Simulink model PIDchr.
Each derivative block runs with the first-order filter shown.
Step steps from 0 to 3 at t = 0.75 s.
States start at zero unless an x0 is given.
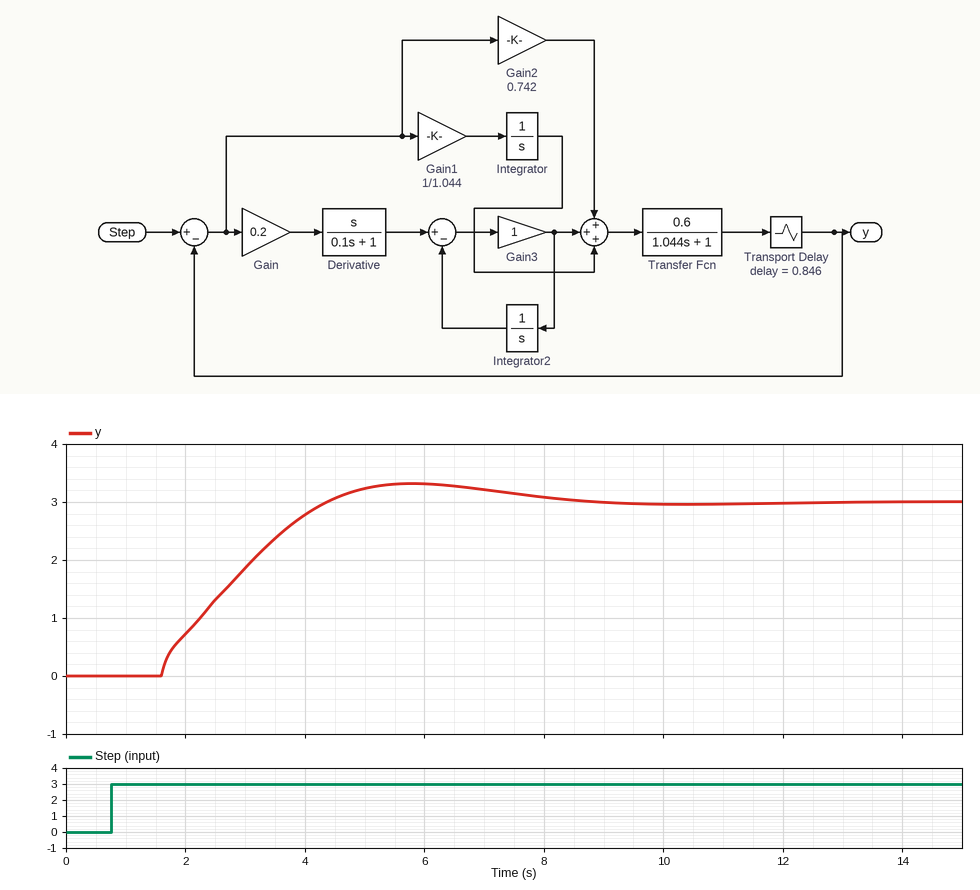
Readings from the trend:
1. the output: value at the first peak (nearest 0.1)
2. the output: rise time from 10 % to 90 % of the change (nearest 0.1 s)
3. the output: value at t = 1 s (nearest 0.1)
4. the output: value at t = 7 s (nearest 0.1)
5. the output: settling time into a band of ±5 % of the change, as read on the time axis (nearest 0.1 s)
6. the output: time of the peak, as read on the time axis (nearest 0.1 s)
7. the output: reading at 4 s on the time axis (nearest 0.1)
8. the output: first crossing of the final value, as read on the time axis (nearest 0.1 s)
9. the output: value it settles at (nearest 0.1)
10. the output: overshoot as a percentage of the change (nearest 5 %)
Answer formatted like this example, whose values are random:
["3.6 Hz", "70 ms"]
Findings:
["3.3", "2.2 s", "0.0", "3.2", "7.5 s", "5.8 s", "2.8", "4.4 s", "3.0", "10 %"]
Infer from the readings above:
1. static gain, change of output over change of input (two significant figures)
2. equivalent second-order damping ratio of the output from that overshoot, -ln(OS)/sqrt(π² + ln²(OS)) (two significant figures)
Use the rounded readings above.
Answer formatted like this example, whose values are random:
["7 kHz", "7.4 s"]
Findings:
["1.0", "0.59"]
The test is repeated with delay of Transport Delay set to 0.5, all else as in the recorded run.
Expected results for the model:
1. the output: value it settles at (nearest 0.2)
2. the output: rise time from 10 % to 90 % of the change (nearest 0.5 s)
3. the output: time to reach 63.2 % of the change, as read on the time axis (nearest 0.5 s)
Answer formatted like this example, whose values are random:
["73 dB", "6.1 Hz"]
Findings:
["3.0", "2.5 s", "3.0 s"]
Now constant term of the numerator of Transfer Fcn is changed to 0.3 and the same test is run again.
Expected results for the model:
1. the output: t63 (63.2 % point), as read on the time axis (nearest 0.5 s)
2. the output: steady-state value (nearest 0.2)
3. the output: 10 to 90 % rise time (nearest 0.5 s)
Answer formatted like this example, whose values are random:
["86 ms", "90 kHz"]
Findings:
["4.5 s", "3.0", "5.0 s"]
